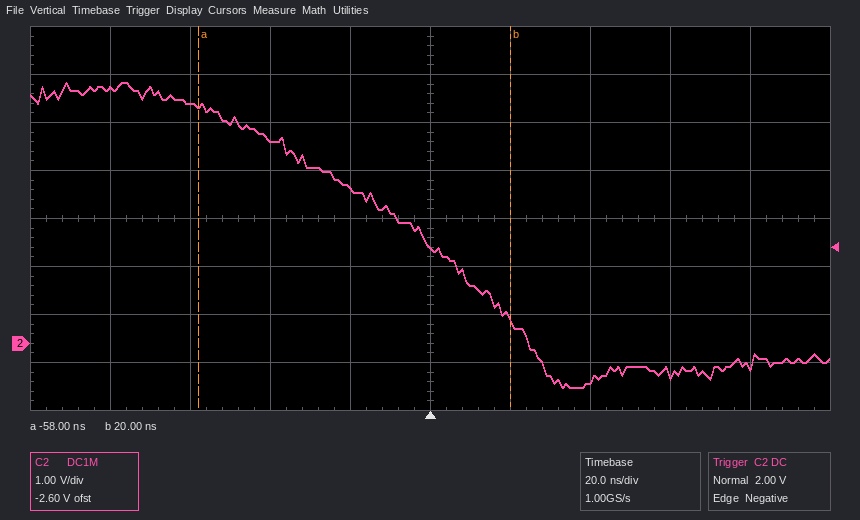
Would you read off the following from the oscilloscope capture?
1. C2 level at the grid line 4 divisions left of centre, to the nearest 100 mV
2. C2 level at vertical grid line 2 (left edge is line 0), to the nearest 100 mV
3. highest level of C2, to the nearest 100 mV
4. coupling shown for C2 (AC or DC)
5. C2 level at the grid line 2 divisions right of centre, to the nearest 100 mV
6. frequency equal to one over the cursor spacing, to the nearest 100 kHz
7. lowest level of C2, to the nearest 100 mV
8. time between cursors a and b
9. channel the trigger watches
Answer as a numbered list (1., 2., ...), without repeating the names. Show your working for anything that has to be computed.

1. 5.3 V
2. 5.0 V
3. 5.4 V
4. DC
5. -800 mV
6. 1 / 78 ns ≈ 12.8 MHz
7. -900 mV
8. 20 ns − (-58 ns) = 78 ns
9. C2
